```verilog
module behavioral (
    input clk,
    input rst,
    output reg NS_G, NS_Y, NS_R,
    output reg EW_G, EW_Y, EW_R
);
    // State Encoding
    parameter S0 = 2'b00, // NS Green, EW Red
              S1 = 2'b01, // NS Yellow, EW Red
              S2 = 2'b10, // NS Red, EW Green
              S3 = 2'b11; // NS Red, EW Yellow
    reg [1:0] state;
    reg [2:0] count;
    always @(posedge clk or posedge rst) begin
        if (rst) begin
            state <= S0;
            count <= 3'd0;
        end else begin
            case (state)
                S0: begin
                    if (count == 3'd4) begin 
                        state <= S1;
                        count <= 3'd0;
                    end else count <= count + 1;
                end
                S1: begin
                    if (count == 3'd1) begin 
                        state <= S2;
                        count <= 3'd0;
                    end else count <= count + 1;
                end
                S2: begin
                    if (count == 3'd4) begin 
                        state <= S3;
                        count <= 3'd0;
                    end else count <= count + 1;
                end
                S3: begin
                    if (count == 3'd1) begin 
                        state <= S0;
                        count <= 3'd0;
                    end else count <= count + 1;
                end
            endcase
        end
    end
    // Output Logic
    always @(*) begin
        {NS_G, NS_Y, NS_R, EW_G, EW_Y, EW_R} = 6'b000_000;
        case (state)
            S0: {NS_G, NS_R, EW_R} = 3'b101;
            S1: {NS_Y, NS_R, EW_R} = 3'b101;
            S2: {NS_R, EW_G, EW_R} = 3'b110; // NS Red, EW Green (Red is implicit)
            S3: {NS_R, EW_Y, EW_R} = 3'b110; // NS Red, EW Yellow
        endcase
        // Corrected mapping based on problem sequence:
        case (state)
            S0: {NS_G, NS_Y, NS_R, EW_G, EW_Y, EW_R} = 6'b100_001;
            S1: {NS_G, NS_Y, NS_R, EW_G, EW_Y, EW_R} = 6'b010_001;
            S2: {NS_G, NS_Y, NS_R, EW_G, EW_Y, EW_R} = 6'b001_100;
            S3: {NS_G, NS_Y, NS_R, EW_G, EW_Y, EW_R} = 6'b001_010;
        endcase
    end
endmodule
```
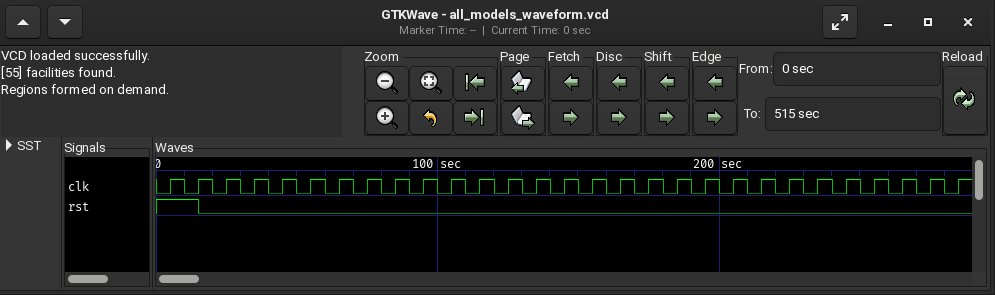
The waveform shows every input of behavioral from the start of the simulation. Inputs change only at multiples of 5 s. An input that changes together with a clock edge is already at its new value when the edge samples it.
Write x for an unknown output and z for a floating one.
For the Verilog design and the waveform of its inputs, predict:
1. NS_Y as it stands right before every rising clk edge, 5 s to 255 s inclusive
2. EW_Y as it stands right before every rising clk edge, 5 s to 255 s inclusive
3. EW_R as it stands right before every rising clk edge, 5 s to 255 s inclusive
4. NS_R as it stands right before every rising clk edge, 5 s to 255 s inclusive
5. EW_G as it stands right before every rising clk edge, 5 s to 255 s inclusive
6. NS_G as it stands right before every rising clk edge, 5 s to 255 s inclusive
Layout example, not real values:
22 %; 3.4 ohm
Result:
0 0 0 0 0 0 1 1 0 0 0 0 0 0 0 0 0 0 0 0 1 1 0 0 0 0; 0 0 0 0 0 0 0 0 0 0 0 0 0 1 1 0 0 0 0 0 0 0 0 0 0 0; 1 1 1 1 1 1 1 1 0 0 0 0 0 0 0 1 1 1 1 1 1 1 0 0 0 0; 0 0 0 0 0 0 0 0 1 1 1 1 1 1 1 0 0 0 0 0 0 0 1 1 1 1; 0 0 0 0 0 0 0 0 1 1 1 1 1 0 0 0 0 0 0 0 0 0 1 1 1 1; 1 1 1 1 1 1 0 0 0 0 0 0 0 0 0 1 1 1 1 1 0 0 0 0 0 0
